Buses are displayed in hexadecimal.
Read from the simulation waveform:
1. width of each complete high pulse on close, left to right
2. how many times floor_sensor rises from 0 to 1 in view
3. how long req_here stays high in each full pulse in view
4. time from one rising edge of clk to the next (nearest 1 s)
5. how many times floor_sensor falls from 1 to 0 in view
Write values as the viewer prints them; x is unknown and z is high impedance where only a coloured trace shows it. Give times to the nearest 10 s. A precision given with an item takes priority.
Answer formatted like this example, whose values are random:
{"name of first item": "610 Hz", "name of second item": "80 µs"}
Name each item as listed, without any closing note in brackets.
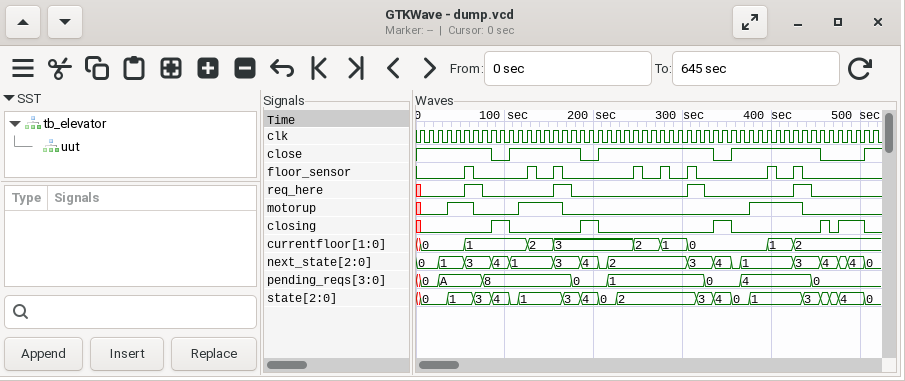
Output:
{"width of each complete high pulse on close, left to right": "80 s, 130 s, 100 s", "how many times floor_sensor rises from 0 to 1 in view": "8", "how long req_here stays high in each full pulse in view": "20 s, 20 s, 20 s, 20 s", "time from one rising edge of clk to the next": "10 s", "how many times floor_sensor falls from 1 to 0 in view": "8"}
